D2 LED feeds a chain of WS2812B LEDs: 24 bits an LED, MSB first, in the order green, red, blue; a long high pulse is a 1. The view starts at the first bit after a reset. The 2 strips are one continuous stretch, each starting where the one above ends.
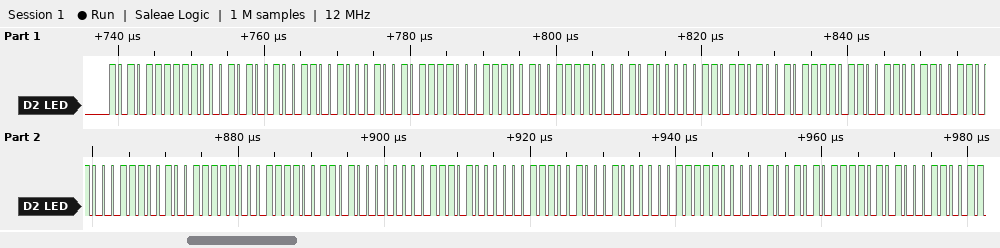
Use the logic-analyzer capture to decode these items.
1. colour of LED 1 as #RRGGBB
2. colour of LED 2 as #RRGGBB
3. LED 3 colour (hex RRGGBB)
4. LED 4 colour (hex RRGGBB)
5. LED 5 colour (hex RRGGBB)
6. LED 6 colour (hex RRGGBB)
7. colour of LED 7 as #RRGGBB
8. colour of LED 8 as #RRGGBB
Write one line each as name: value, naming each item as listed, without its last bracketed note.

colour of LED 1 as #RRGGBB: #C5AF26
colour of LED 2 as #RRGGBB: #BC4472
LED 3 colour: #50786D
LED 4 colour: #662F66
LED 5 colour: #4F8E8F
LED 6 colour: #0334A0
colour of LED 7 as #RRGGBB: #20727C
colour of LED 8 as #RRGGBB: #BD1246
